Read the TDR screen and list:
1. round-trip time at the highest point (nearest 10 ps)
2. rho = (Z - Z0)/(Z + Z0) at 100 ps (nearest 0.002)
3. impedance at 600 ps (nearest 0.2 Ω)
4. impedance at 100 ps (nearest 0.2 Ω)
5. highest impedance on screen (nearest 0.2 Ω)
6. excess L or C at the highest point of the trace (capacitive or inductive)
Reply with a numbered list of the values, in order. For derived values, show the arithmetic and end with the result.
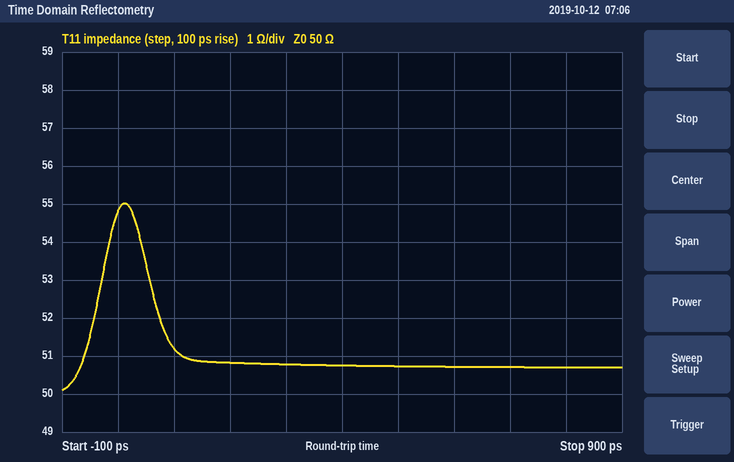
1. 10 ps
2. (51.2 − 50)/(51.2 + 50) ≈ +0.012
3. 50.8 Ω
4. 51.2 Ω
5. 55.0 Ω
6. inductive
